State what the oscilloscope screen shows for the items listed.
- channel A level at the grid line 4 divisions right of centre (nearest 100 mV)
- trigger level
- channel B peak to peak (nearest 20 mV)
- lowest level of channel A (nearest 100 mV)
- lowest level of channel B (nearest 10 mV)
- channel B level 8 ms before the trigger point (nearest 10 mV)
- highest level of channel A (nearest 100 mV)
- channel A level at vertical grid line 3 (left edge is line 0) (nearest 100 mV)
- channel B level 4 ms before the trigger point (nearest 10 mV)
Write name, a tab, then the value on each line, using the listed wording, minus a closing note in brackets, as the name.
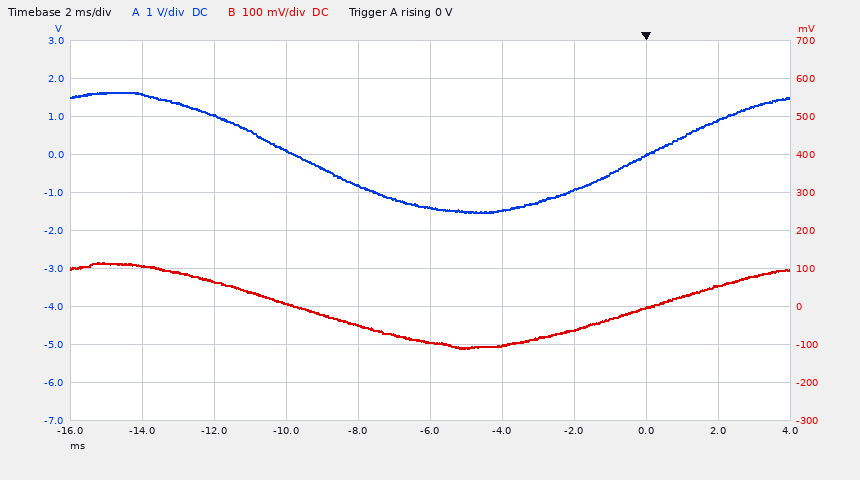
channel A level at the grid line 4 divisions right of centre	900 mV
trigger level	0 V
channel B peak to peak	220 mV
lowest level of channel A	-1.5 V
lowest level of channel B	-110 mV
channel B level 8 ms before the trigger point	-50 mV
highest level of channel A	1.6 V
channel A level at vertical grid line 3 (left edge is line 0)	100 mV
channel B level 4 ms before the trigger point	-100 mV
